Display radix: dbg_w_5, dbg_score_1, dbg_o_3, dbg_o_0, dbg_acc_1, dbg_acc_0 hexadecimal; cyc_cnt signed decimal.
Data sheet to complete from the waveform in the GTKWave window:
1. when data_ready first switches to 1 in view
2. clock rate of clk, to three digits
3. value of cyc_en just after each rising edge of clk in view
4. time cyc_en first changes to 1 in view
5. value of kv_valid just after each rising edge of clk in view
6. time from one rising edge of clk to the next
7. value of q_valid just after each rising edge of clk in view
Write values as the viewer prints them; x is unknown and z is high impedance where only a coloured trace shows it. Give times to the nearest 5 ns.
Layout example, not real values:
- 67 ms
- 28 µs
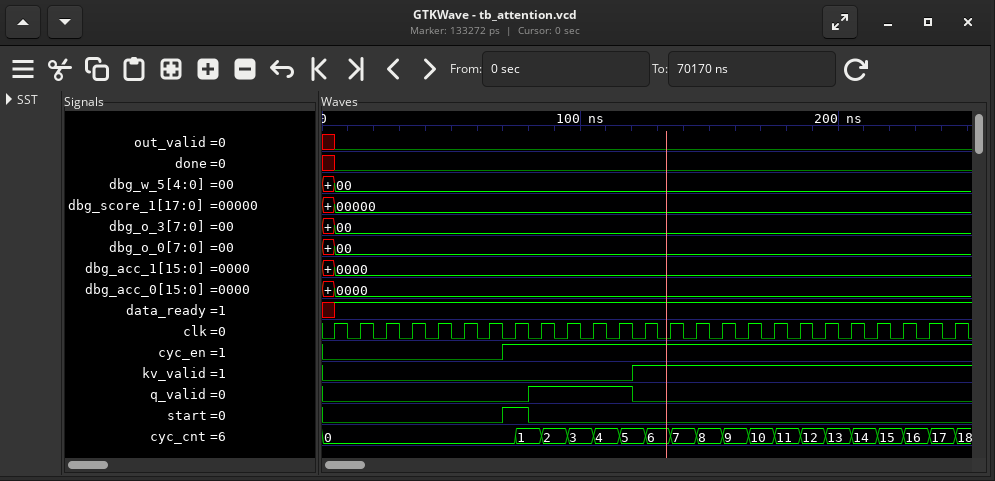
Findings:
- 5 ns
- 100 MHz
- 0 0 0 0 0 0 0 1 1 1 1 1 1 1 1 1 1 1 1 1 1 1 1 1 1
- 70 ns
- 0 0 0 0 0 0 0 0 0 0 0 0 1 1 1 1 1 1 1 1 1 1 1 1 1
- 10 ns
- 0 0 0 0 0 0 0 0 1 1 1 1 0 0 0 0 0 0 0 0 0 0 0 0 0
